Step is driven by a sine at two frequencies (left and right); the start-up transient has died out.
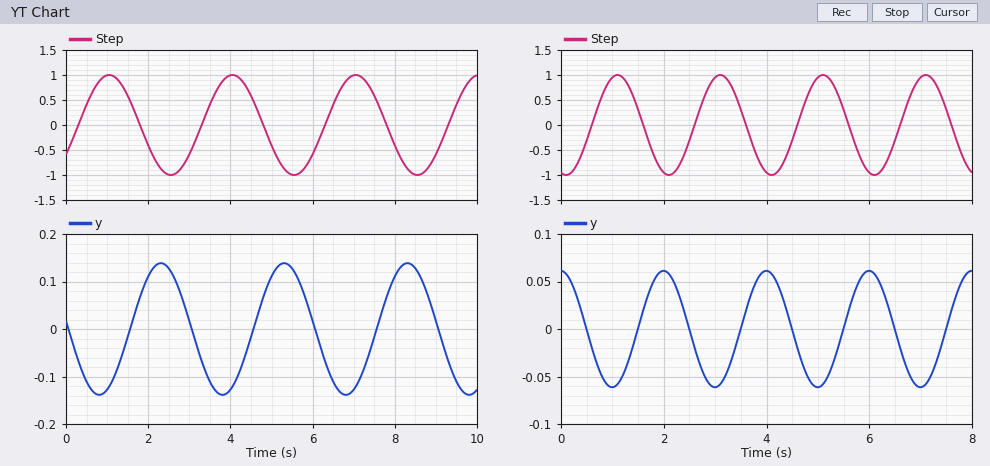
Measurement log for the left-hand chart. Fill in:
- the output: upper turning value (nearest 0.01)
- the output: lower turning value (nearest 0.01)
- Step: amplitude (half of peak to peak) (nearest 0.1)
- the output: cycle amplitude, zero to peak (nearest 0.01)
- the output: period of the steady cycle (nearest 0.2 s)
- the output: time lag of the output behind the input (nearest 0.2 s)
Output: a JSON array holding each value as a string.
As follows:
["0.14", "-0.14", "1.0", "0.14", "3.0 s", "1.2 s"]
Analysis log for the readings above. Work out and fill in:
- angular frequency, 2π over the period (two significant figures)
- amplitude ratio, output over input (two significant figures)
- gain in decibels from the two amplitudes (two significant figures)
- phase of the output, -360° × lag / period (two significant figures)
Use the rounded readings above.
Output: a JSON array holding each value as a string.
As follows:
["2.1 rad/s", "0.14", "-17 dB", "-140°"]
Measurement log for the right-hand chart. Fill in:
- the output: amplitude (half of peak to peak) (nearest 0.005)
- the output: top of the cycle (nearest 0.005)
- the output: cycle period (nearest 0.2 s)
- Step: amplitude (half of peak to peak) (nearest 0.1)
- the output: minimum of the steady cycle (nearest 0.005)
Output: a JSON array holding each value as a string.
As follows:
["0.060", "0.060", "2.0 s", "1.0", "-0.060"]
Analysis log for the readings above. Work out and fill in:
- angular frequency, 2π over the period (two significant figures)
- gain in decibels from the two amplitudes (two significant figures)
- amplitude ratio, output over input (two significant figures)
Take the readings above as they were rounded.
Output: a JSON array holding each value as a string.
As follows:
["3.1 rad/s", "-24 dB", "0.060"]
